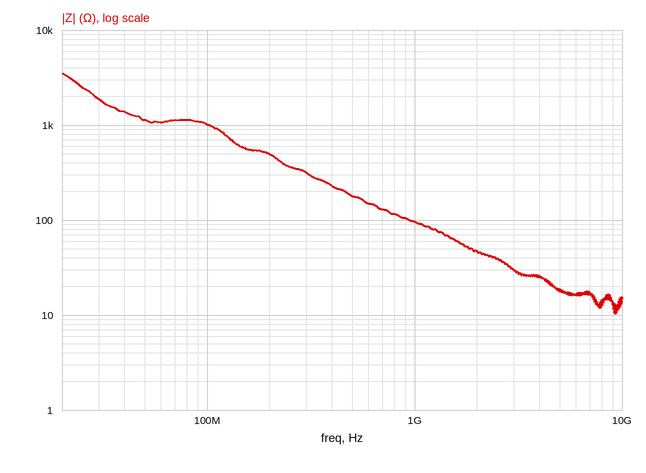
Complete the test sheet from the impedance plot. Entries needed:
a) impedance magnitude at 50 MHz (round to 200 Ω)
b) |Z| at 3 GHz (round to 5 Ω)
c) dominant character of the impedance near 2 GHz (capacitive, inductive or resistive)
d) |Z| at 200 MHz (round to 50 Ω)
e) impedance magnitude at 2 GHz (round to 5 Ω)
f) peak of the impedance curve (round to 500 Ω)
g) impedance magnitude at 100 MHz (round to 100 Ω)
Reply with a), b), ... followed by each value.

a) 1.2 kΩ
b) 30 Ω
c) capacitive
d) 500 Ω
e) 45 Ω
f) 3.5 kΩ
g) 1.0 kΩ
